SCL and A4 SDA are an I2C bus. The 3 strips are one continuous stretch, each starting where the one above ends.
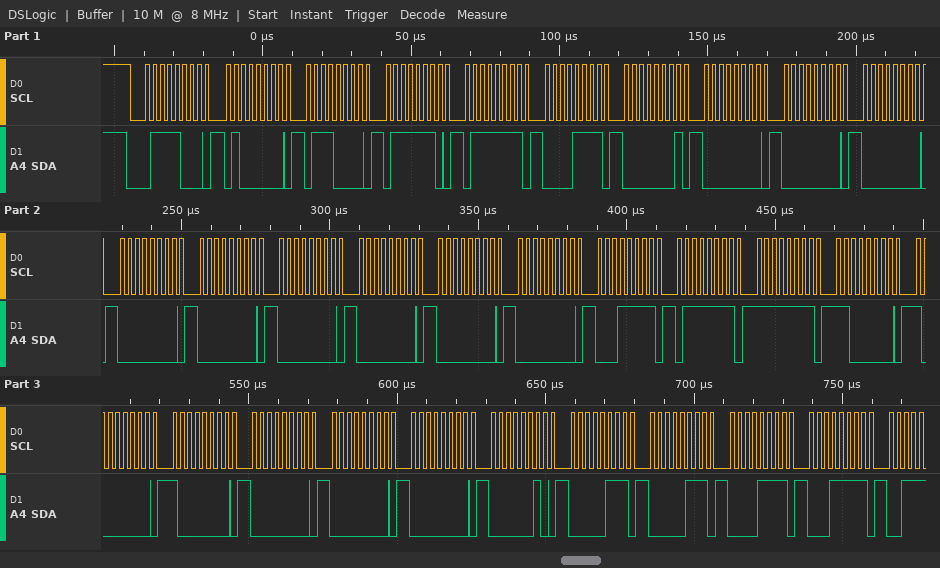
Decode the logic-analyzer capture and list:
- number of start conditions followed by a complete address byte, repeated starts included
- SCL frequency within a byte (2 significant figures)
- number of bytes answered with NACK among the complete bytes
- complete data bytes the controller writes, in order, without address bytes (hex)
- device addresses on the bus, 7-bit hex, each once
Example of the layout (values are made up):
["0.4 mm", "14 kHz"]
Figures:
["1", "400 kHz", "0", "40 70 7E 7F 0F 01 00 00 00 00 00 00 00 00 00 1F 7F FF C0 80 80 00 00 00 02 07 07 0F 1F", "0x3C"]
